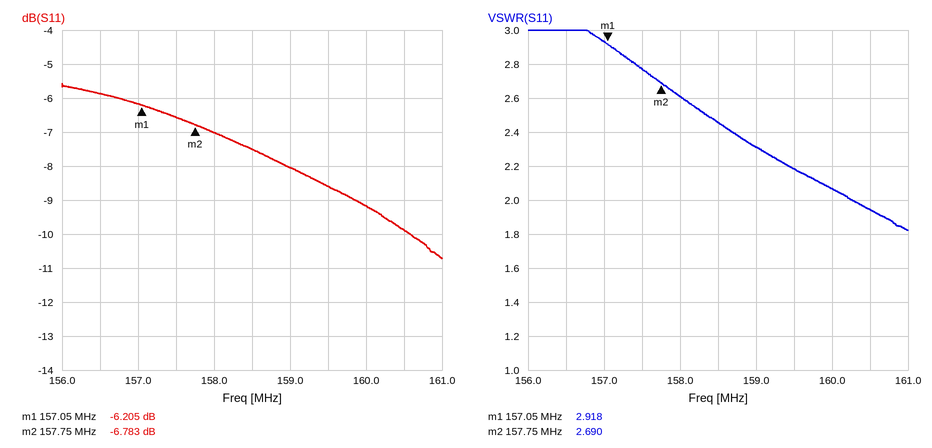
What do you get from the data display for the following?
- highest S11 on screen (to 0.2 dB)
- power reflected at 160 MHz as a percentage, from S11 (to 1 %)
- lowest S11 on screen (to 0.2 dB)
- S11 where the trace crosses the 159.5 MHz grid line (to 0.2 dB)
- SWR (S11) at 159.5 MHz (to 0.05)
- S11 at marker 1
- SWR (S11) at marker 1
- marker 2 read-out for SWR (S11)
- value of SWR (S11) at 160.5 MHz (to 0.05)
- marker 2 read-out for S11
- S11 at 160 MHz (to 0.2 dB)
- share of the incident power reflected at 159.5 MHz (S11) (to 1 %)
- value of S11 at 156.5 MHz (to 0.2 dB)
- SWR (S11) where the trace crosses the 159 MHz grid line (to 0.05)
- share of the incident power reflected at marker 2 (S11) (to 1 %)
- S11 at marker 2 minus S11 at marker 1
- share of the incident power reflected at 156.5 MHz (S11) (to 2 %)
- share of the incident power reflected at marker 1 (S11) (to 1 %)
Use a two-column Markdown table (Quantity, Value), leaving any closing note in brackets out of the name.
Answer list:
| Quantity | Value |
|---|---|
| highest S11 on screen | -5.6 dB |
| power reflected at 160 MHz as a percentage, from S11 | 12 % |
| lowest S11 on screen | -10.8 dB |
| S11 where the trace crosses the 159.5 MHz grid line | -8.6 dB |
| SWR (S11) at 159.5 MHz | 2.20 |
| S11 at marker 1 | -6.205 dB |
| SWR (S11) at marker 1 | 2.918 |
| marker 2 read-out for SWR | 2.690 |
| value of SWR (S11) at 160.5 MHz | 1.95 |
| marker 2 read-out for S11 | -6.783 dB |
| S11 at 160 MHz | -9.2 dB |
| share of the incident power reflected at 159.5 MHz (S11) | 14 % |
| value of S11 at 156.5 MHz | -5.8 dB |
| SWR (S11) where the trace crosses the 159 MHz grid line | 2.30 |
| share of the incident power reflected at marker 2 (S11) | 21 % |
| S11 at marker 2 minus S11 at marker 1 | -0.578 dB |
| share of the incident power reflected at 156.5 MHz (S11) | 26 % |
| share of the incident power reflected at marker 1 (S11) | 24 % |
